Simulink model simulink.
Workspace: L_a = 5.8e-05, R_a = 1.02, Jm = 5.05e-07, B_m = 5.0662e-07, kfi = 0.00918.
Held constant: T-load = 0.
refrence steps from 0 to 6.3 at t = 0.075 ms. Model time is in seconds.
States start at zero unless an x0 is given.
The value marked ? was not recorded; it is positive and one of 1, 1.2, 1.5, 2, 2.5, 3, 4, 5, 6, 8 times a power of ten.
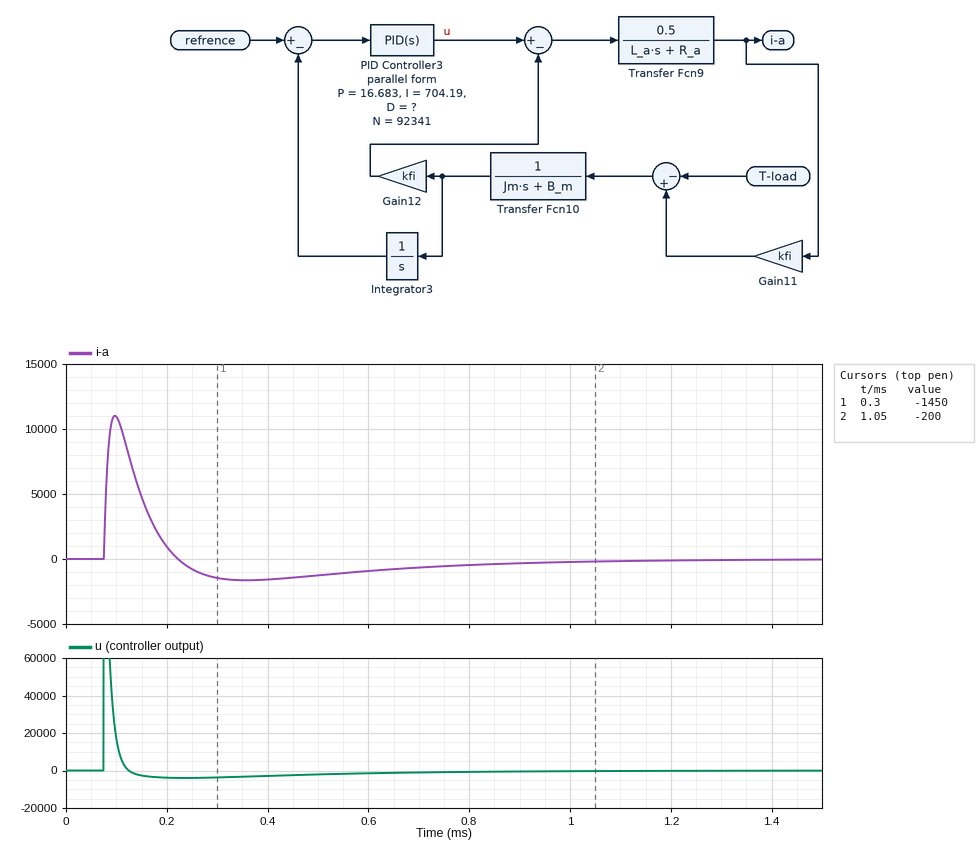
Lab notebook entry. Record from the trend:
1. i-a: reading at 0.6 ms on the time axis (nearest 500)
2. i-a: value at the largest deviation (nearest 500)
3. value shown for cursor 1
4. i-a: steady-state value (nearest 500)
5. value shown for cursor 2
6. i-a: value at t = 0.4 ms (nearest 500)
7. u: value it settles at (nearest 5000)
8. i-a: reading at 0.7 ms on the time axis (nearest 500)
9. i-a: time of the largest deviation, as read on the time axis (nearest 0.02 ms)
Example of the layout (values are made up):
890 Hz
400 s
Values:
-1000
11000
-1450
0
-200
-1500
0
-500
0.10 ms
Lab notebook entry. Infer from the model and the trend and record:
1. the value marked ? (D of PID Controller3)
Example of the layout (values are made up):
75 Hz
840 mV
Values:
0.3
